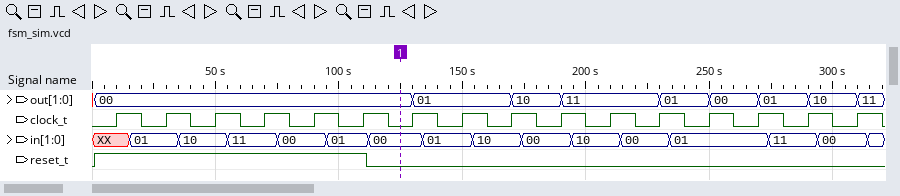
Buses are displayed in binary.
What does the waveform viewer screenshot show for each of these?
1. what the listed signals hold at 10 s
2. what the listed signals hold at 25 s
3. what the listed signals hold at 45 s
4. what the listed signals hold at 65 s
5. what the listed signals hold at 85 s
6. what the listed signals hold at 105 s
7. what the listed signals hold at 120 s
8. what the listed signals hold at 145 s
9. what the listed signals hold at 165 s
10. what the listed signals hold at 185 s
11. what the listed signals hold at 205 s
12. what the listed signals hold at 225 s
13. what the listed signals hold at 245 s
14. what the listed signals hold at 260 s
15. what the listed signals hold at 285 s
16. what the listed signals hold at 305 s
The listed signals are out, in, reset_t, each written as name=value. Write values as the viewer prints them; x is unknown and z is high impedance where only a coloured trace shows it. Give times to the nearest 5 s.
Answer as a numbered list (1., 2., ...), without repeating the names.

1. out=00, in=XX, reset_t=1
2. out=00, in=01, reset_t=1
3. out=00, in=10, reset_t=1
4. out=00, in=11, reset_t=1
5. out=00, in=00, reset_t=1
6. out=00, in=01, reset_t=1
7. out=00, in=00, reset_t=0
8. out=01, in=01, reset_t=0
9. out=01, in=10, reset_t=0
10. out=10, in=00, reset_t=0
11. out=11, in=10, reset_t=0
12. out=11, in=00, reset_t=0
13. out=01, in=01, reset_t=0
14. out=00, in=01, reset_t=0
15. out=01, in=11, reset_t=0
16. out=10, in=00, reset_t=0
